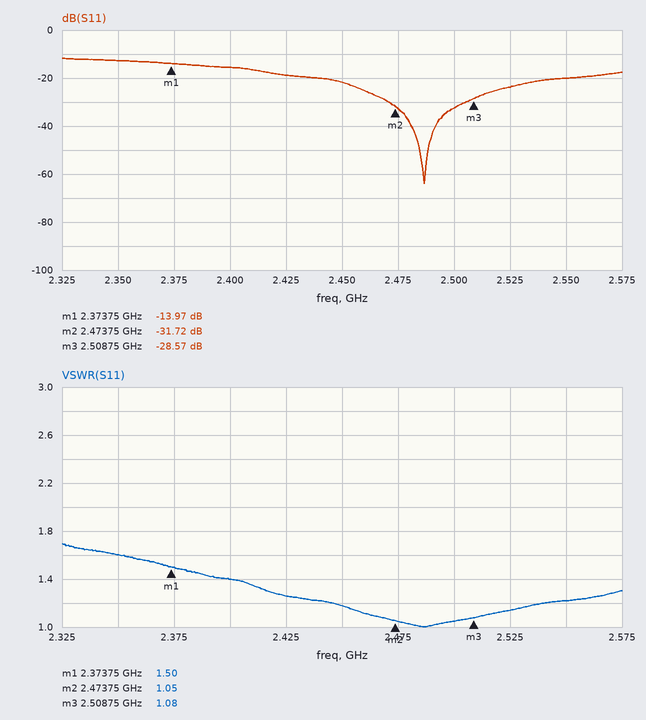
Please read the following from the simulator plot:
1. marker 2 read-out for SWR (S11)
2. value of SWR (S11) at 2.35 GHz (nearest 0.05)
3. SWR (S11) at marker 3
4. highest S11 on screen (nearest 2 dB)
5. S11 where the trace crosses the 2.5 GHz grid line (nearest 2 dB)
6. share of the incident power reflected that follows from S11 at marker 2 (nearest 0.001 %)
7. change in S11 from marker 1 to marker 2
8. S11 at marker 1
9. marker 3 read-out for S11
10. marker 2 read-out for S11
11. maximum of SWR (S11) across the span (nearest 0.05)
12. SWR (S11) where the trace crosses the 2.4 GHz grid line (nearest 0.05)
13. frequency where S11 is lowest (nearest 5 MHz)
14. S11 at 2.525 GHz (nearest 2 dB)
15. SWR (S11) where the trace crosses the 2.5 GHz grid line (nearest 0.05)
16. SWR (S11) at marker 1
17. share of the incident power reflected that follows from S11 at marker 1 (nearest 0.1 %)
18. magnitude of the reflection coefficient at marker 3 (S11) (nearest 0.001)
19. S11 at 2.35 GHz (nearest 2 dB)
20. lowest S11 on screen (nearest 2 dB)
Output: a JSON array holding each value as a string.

["1.05", "1.60", "1.08", "-12 dB", "-32 dB", "0.067 %", "-17.75 dB", "-13.97 dB", "-28.57 dB", "-31.72 dB", "1.70", "1.40", "2.485 GHz", "-24 dB", "1.05", "1.50", "4.0 %", "0.037", "-12 dB", "-64 dB"]
